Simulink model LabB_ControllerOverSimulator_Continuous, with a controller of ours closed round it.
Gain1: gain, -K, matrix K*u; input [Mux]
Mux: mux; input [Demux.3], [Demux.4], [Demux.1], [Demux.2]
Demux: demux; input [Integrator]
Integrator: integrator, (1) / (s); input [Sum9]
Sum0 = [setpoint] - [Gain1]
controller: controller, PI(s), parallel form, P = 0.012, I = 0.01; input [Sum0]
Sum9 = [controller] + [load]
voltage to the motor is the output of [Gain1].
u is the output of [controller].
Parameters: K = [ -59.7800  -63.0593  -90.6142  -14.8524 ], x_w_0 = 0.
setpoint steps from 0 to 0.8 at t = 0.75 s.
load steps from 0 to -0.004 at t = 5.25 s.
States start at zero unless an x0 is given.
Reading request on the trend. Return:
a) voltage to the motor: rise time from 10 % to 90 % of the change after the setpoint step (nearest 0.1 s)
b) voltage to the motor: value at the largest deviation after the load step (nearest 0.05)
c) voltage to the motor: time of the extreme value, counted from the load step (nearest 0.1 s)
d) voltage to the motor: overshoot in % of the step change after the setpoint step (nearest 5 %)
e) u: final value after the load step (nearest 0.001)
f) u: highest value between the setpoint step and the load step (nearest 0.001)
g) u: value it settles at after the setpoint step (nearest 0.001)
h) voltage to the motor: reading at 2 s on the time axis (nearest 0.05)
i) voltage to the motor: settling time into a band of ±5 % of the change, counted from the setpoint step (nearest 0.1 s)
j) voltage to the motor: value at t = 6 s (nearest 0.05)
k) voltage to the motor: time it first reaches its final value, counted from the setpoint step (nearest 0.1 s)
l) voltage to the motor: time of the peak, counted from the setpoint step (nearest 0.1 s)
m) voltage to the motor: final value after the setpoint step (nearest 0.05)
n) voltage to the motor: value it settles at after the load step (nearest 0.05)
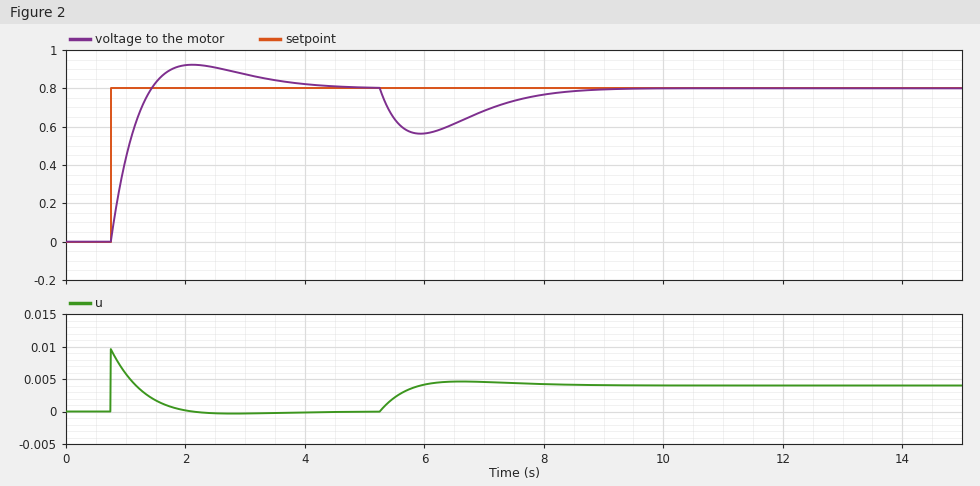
0.5 s
0.55
0.7 s
15 %
0.004
0.010
0.000
0.90
2.8 s
0.55
0.7 s
1.4 s
0.80
0.80
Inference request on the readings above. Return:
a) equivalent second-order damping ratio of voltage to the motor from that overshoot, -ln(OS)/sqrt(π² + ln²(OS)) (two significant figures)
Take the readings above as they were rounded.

0.52
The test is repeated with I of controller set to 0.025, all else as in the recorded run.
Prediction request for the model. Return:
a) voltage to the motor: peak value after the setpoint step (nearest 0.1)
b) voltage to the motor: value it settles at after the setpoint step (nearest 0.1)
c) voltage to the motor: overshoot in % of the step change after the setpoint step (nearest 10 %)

1.0
0.8
30 %
